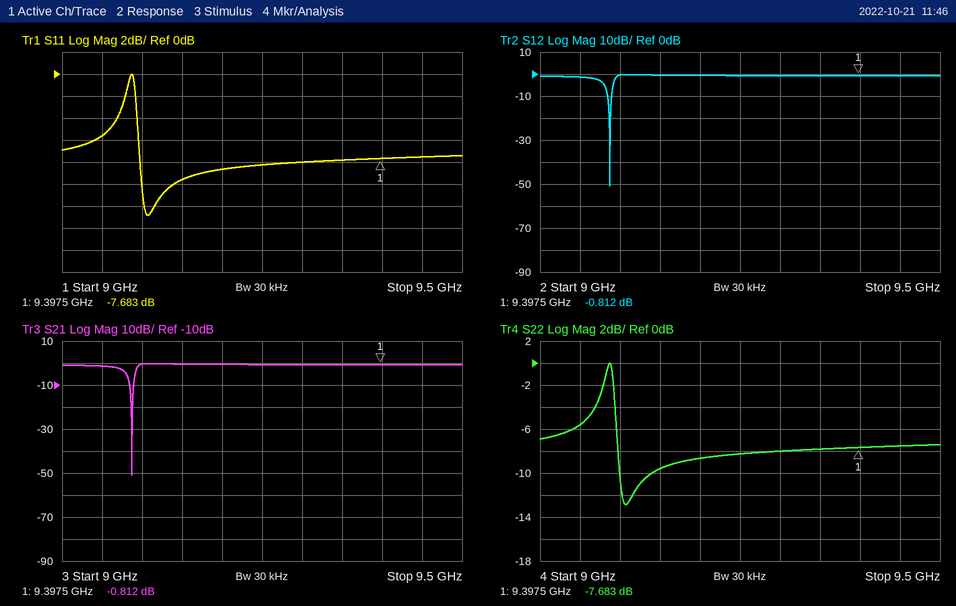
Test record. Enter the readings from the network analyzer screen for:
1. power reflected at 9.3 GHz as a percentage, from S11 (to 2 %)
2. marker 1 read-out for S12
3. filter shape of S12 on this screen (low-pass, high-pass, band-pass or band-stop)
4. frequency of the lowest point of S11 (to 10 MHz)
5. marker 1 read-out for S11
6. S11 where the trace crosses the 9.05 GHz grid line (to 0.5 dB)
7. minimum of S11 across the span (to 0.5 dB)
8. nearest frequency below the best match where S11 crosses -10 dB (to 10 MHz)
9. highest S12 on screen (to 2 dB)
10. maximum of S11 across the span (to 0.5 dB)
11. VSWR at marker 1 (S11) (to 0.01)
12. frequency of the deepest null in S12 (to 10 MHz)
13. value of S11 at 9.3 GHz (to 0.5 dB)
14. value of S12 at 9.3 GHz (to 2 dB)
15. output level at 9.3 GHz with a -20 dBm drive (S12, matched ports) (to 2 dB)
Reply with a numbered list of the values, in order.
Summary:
1. 16 %
2. -0.812 dB
3. band-stop
4. 9.11 GHz
5. -7.683 dB
6. -5.5 dB
7. -13.0 dB
8. 9.10 GHz
9. 0 dB
10. 0.0 dB
11. 2.41
12. 9.09 GHz
13. -8.0 dB
14. 0 dB
15. -20 dBm
